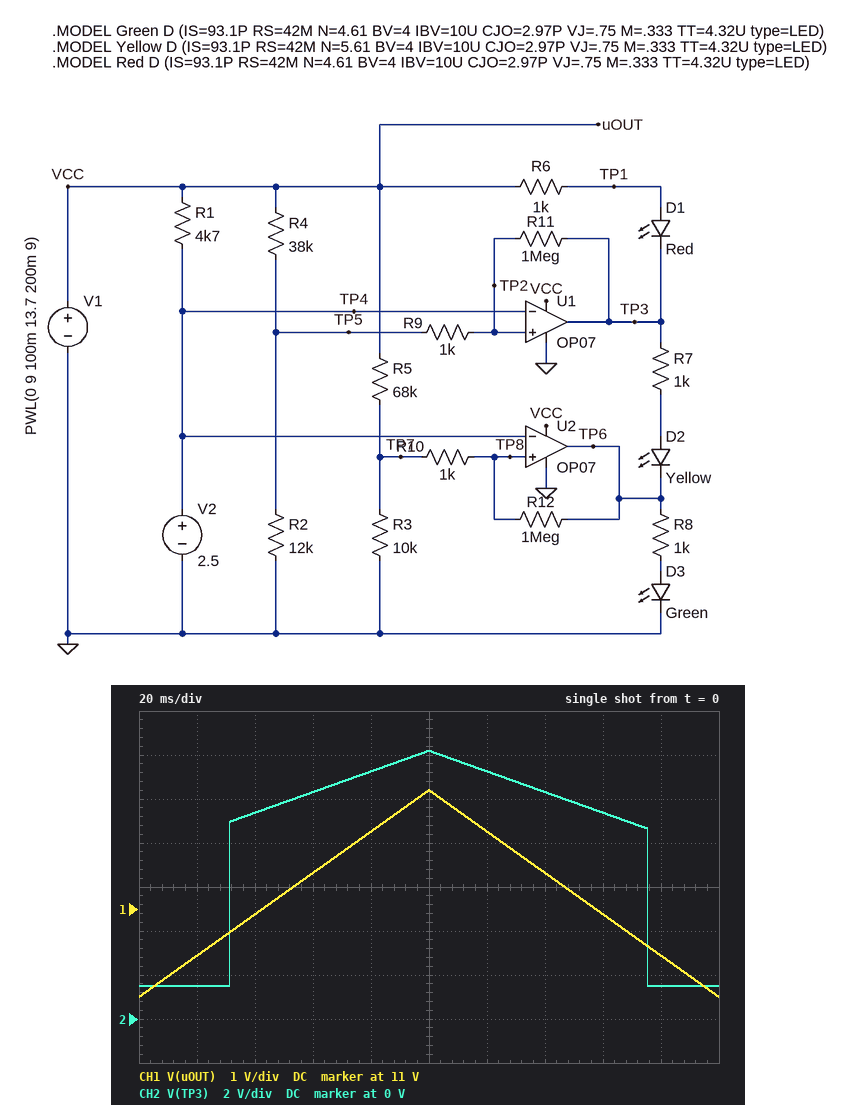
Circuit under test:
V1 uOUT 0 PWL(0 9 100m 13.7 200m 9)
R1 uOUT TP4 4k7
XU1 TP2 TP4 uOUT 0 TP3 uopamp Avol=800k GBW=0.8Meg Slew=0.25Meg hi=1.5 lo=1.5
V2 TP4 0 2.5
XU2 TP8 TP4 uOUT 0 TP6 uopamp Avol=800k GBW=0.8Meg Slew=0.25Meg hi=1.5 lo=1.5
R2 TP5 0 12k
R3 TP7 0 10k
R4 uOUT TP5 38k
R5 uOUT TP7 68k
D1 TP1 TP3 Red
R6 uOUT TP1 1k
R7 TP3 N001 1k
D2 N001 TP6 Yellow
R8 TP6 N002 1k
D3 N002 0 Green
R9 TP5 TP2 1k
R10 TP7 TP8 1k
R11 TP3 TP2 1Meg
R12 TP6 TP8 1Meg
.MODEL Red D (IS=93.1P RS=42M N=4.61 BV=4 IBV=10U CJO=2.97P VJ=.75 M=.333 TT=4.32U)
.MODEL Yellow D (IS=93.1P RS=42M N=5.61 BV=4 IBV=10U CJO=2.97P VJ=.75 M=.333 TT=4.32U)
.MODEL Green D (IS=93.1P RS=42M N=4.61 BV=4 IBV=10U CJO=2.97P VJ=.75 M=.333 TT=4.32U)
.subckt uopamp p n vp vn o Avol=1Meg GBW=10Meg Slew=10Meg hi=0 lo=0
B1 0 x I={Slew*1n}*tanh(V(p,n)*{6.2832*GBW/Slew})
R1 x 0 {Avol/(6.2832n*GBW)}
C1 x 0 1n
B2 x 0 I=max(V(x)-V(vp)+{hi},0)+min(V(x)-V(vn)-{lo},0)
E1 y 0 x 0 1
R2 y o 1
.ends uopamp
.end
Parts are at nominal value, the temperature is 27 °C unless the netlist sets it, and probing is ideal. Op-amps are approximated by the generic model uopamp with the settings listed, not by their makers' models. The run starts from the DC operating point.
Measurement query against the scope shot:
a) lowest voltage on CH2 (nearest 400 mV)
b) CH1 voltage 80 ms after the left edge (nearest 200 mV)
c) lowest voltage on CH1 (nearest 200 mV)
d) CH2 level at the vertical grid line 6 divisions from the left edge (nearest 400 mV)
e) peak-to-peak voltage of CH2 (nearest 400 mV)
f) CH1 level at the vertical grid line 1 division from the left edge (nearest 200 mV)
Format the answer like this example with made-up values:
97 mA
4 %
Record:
1.6 V
12.8 V
9.0 V
11.2 V
10.8 V
10.0 V
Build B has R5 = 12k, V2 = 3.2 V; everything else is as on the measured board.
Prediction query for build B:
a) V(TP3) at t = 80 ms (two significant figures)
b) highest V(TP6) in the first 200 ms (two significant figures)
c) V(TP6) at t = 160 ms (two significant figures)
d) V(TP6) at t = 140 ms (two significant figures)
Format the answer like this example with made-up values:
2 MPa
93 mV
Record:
1.5 V
12 V
9.4 V
10 V
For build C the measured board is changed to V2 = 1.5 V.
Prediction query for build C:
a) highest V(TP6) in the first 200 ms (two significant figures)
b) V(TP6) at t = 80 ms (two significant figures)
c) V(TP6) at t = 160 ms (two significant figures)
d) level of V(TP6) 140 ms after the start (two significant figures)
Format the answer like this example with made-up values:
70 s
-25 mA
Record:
12 V
11 V
1.5 V
10 V
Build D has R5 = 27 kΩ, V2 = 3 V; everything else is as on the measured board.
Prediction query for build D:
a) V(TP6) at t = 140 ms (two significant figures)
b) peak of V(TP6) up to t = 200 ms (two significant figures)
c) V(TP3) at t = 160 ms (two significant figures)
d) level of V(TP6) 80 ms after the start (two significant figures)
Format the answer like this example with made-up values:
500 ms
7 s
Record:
10 V
12 V
1.5 V
11 V
